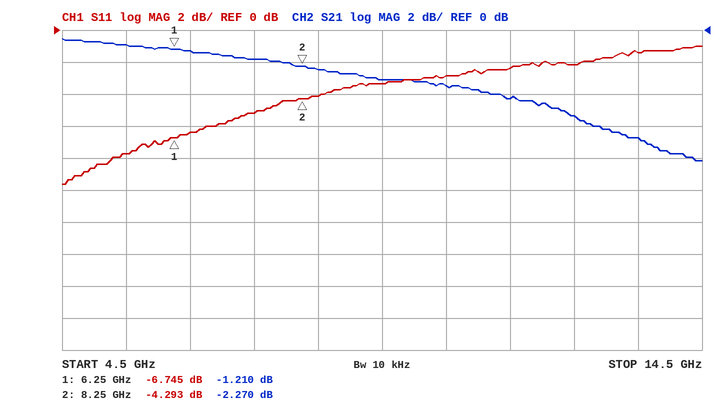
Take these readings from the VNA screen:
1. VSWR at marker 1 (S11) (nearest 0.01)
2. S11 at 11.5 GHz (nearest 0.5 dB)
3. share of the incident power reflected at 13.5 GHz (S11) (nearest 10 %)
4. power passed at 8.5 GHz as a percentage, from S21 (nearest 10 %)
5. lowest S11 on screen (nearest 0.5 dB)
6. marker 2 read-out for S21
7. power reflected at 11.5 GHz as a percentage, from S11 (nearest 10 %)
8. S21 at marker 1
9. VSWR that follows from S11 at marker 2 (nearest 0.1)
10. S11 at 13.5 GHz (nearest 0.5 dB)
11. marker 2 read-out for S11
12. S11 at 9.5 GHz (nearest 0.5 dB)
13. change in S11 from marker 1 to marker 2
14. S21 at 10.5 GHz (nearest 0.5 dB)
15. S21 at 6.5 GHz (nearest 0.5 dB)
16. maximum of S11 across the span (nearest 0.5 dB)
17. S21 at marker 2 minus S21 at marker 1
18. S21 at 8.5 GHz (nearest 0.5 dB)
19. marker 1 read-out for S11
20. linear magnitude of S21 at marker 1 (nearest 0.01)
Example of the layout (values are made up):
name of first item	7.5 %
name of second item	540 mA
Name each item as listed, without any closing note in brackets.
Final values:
VSWR at marker 1 (S11)	2.70
S11 at 11.5 GHz	-2.5 dB
share of the incident power reflected at 13.5 GHz (S11)	70 %
power passed at 8.5 GHz as a percentage, from S21	60 %
lowest S11 on screen	-9.5 dB
marker 2 read-out for S21	-2.270 dB
power reflected at 11.5 GHz as a percentage, from S11	60 %
S21 at marker 1	-1.210 dB
VSWR that follows from S11 at marker 2	4.1
S11 at 13.5 GHz	-1.5 dB
marker 2 read-out for S11	-4.293 dB
S11 at 9.5 GHz	-3.5 dB
change in S11 from marker 1 to marker 2	2.452 dB
S21 at 10.5 GHz	-3.5 dB
S21 at 6.5 GHz	-1.5 dB
maximum of S11 across the span	-1.0 dB
S21 at marker 2 minus S21 at marker 1	-1.060 dB
S21 at 8.5 GHz	-2.5 dB
marker 1 read-out for S11	-6.745 dB
linear magnitude of S21 at marker 1	0.87
